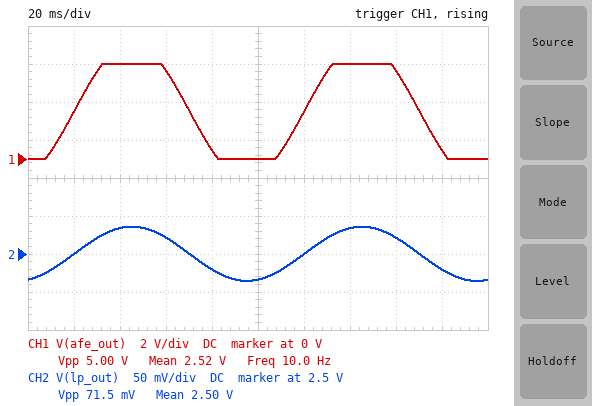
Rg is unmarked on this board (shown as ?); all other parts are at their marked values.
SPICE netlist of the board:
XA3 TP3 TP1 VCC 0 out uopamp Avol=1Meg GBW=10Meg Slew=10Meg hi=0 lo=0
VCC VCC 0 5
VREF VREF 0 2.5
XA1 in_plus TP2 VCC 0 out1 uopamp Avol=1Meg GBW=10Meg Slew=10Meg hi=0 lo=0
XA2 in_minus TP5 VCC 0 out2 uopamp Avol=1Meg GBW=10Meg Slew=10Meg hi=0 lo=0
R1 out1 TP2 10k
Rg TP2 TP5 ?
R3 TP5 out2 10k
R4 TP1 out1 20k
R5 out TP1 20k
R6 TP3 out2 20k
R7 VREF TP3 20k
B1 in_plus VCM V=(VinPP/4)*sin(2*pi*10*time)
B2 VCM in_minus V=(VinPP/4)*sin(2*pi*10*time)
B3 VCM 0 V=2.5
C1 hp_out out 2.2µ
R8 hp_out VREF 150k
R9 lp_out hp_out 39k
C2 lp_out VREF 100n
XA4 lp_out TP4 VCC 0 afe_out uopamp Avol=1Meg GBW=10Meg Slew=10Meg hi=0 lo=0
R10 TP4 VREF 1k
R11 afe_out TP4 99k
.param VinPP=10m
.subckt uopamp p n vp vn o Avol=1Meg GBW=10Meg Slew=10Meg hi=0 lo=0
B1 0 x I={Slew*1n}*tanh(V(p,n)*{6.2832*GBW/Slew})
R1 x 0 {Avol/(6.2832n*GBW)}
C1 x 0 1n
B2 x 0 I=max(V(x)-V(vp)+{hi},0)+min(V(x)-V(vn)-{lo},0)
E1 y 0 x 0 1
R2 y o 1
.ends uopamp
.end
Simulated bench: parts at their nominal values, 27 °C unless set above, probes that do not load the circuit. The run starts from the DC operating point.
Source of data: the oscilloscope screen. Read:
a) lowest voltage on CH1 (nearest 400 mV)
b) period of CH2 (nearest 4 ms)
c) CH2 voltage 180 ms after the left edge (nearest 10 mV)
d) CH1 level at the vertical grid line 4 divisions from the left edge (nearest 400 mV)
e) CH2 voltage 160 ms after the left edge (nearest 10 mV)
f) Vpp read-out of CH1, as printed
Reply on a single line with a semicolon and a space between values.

0 V; 100 ms; 2.48 V; 400 mV; 2.52 V; 5.00 V
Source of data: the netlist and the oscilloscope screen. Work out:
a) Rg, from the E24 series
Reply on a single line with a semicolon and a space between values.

3 kΩ
